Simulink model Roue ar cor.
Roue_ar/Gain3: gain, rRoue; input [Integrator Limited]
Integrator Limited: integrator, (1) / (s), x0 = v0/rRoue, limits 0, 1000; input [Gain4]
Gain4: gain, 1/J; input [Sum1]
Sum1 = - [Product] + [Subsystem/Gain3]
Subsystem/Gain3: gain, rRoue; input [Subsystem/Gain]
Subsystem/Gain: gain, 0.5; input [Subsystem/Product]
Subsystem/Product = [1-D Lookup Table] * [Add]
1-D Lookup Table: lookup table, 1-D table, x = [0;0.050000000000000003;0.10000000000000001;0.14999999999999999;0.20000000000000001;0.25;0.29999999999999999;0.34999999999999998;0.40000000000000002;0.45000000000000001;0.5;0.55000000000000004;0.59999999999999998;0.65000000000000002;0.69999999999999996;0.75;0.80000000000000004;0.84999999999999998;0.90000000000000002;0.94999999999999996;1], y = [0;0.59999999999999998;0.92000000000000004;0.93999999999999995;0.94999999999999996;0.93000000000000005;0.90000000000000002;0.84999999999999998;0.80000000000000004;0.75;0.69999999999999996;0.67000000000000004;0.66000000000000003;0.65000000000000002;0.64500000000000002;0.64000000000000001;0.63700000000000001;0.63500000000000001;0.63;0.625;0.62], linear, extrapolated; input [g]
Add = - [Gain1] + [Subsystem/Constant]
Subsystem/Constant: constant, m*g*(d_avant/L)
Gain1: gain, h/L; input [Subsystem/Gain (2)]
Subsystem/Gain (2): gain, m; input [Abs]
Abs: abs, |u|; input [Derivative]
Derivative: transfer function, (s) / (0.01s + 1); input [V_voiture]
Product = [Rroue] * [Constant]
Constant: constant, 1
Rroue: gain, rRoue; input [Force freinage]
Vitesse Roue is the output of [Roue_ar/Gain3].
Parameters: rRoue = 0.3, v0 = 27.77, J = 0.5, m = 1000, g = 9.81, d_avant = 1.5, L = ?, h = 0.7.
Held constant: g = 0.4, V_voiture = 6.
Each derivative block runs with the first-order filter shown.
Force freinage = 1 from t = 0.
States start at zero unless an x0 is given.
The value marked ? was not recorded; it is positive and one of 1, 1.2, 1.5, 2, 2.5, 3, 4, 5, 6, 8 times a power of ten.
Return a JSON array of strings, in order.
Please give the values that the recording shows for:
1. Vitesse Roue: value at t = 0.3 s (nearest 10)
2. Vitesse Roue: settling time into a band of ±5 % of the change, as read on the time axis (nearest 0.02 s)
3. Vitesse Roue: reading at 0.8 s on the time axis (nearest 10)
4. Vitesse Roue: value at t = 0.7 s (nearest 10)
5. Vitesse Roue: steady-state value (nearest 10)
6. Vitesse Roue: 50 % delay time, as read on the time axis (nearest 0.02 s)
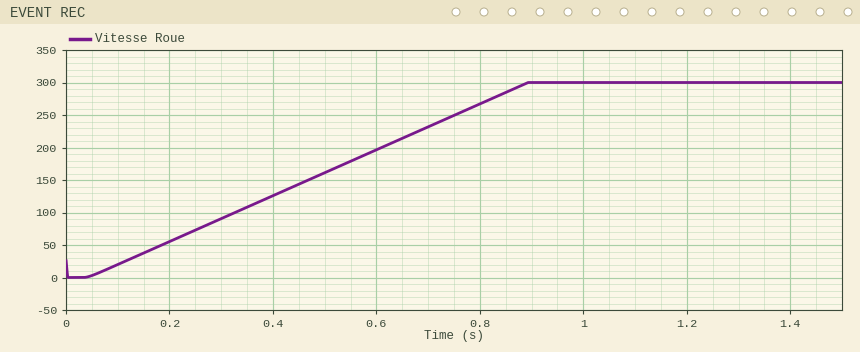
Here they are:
["90", "0.86 s", "270", "230", "300", "0.50 s"]
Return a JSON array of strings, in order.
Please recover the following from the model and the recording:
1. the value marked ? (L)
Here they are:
["3"]
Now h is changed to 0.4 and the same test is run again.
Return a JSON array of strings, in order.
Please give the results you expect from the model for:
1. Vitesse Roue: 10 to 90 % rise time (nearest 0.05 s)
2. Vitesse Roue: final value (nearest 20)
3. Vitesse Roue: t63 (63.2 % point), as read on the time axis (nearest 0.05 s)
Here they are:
["0.60 s", "300", "0.60 s"]
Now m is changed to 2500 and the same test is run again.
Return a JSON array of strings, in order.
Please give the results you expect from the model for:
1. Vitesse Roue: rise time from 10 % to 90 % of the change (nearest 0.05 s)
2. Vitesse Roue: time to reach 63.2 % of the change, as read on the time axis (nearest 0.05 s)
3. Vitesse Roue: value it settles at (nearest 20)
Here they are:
["0.25 s", "0.25 s", "300"]
